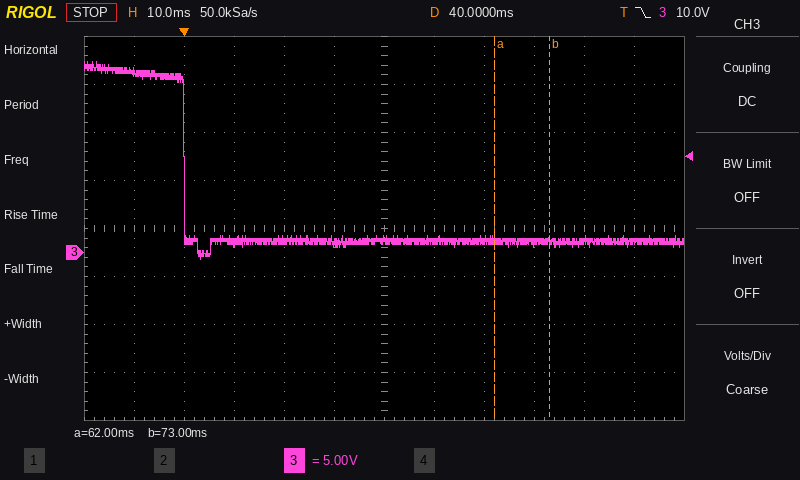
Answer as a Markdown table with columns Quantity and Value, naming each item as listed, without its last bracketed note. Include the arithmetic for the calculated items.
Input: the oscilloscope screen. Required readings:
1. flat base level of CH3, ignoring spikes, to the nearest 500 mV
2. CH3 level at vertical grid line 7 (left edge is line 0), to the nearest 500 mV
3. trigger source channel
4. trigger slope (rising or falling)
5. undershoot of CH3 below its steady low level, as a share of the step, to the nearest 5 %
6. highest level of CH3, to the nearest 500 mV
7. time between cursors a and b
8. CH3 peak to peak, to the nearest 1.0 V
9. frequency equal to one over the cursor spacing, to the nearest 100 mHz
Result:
| Quantity | Value |
|---|---|
| flat base level of CH3, ignoring spikes, to the nearest 500 mV | 1.0 V |
| CH3 level at vertical grid line 7 (left edge is line 0), to the nearest 500 mV | 1.0 V |
| trigger source channel | CH3 |
| trigger slope | falling |
| undershoot of CH3 below its steady low level, as a share of the step, to the nearest 5 % | 10 % |
| highest level of CH3, to the nearest 500 mV | 20.0 V |
| time between cursors a and b | 73 ms − (62 ms) = 11 ms |
| CH3 peak to peak, to the nearest 1.0 V | 21.0 V |
| frequency equal to one over the cursor spacing, to the nearest 100 mHz | 1 / 11 ms ≈ 90.9 Hz |
